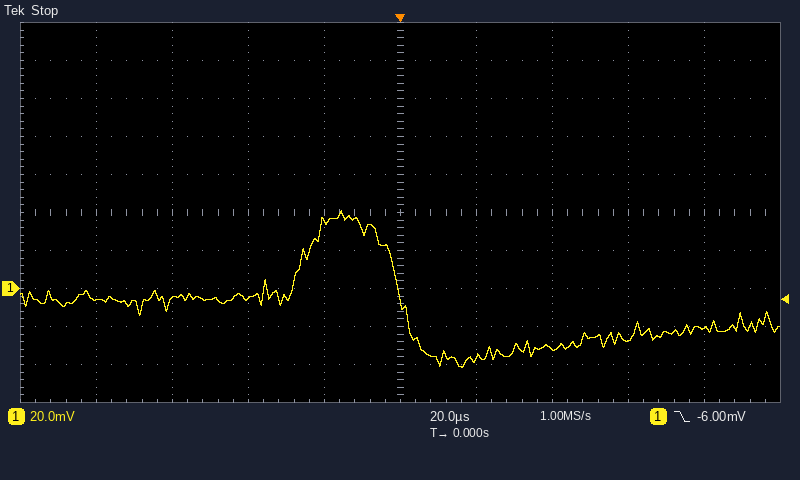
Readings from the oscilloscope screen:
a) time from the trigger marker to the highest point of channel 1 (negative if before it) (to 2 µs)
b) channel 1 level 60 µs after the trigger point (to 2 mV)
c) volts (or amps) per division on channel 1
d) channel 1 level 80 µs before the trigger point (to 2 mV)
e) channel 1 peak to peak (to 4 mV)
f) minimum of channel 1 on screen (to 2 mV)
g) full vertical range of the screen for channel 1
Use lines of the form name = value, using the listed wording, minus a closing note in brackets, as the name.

time from the trigger marker to the highest point of channel 1 (negative if before it) = -16 µs
channel 1 level 60 µs after the trigger point = -26 mV
volts (or amps) per division on channel 1 = 20 mV
channel 1 level 80 µs before the trigger point = -6 mV
channel 1 peak to peak = 84 mV
minimum of channel 1 on screen = -42 mV
full vertical range of the screen for channel 1 = 200 mV
